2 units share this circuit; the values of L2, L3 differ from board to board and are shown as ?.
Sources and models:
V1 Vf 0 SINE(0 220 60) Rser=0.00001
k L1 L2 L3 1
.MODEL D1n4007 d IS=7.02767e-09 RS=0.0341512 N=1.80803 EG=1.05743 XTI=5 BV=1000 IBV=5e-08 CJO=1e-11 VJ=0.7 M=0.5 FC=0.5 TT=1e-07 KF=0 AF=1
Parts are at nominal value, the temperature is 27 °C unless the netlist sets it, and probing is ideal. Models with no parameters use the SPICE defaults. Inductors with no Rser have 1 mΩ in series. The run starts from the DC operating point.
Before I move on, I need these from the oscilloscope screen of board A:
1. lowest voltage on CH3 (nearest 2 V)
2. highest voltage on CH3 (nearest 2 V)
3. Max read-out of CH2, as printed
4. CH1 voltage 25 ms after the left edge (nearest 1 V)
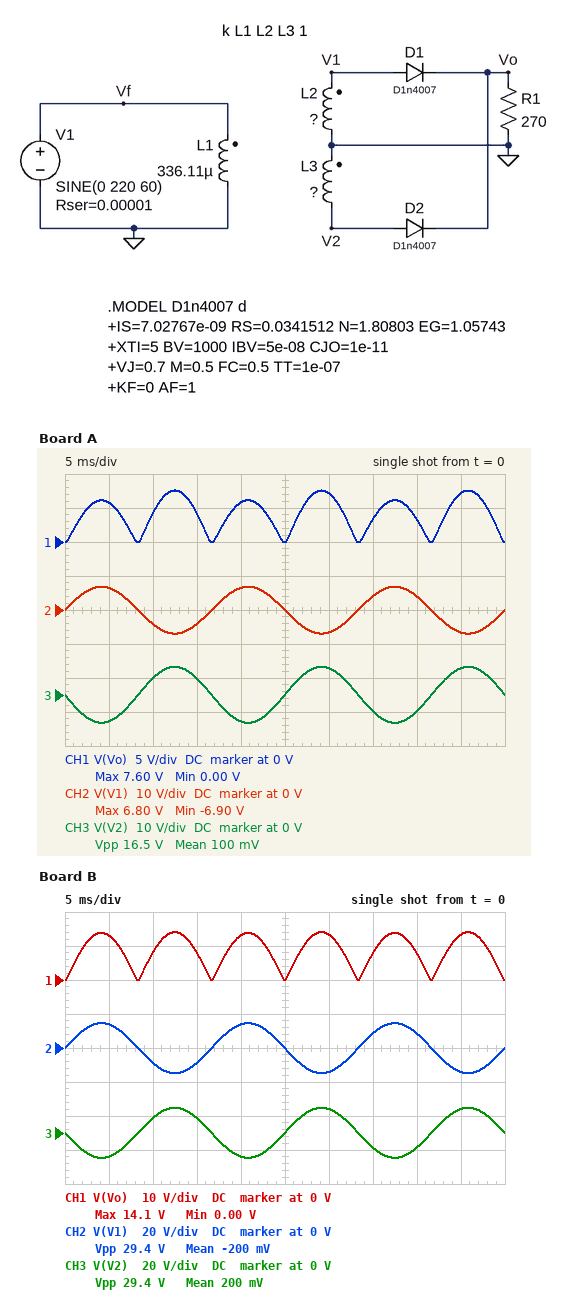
-8 V
8 V
6.80 V
0 V
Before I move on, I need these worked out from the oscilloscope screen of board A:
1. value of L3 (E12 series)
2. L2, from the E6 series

470 nH
330 nH
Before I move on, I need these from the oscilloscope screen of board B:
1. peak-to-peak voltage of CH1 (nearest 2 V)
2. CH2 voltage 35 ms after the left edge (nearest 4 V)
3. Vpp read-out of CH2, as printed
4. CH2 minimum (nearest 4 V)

14 V
8 V
29.4 V
-16 V
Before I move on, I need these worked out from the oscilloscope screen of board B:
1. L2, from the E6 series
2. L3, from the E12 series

1.5 µH
1.5 µH
